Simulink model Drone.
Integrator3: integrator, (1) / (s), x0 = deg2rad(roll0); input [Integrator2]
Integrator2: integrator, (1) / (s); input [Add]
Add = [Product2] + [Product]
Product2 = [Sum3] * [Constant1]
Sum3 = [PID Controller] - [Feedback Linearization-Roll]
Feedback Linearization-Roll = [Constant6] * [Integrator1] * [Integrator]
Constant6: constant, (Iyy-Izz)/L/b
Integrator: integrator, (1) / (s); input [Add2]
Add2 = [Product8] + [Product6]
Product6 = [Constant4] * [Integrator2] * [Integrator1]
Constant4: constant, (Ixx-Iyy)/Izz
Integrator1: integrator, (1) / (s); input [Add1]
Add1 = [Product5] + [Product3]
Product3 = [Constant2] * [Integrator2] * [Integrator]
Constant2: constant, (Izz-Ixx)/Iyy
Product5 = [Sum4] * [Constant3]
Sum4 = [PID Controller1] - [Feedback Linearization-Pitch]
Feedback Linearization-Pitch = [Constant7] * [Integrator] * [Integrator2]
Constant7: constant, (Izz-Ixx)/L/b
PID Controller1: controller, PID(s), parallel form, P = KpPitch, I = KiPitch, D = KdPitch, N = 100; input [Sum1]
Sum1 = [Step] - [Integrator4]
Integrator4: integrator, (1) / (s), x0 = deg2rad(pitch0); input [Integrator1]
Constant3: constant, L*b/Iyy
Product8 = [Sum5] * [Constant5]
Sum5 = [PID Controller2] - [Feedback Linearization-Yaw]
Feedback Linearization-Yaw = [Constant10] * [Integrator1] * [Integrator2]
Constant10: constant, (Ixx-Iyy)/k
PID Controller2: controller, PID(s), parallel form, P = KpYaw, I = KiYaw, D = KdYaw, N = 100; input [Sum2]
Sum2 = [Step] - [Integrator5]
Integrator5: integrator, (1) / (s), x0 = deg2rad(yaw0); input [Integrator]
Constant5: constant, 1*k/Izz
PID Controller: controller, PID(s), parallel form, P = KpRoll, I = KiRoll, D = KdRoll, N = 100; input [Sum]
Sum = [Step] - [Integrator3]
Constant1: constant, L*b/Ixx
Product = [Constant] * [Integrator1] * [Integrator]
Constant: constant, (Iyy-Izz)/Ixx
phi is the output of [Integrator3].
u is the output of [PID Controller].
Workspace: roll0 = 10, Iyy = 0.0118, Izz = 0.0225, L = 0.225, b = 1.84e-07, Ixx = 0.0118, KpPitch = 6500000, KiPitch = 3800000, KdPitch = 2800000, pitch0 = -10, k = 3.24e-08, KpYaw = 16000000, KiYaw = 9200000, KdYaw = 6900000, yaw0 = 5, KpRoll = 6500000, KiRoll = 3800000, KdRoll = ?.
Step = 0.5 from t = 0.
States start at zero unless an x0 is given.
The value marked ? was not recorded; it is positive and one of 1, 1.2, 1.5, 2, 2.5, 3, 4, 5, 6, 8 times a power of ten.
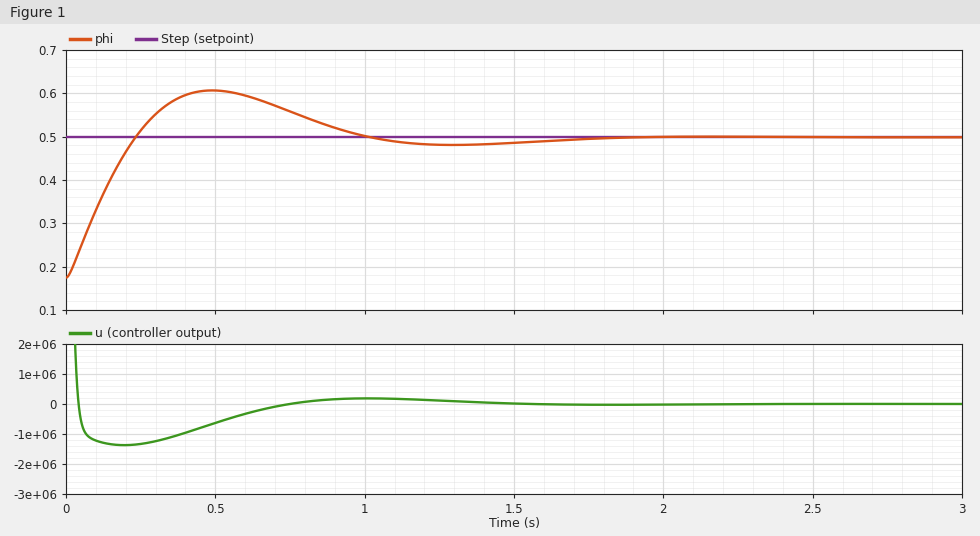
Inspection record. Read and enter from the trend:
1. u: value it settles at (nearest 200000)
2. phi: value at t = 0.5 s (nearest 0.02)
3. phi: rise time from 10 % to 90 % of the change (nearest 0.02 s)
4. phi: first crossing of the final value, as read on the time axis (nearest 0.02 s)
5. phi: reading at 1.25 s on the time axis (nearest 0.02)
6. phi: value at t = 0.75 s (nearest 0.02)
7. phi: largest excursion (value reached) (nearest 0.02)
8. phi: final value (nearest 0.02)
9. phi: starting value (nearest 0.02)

0
0.60
0.18 s
0.24 s
0.48
0.56
0.60
0.50
0.18
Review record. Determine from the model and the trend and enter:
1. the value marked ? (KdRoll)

1.5e+06
